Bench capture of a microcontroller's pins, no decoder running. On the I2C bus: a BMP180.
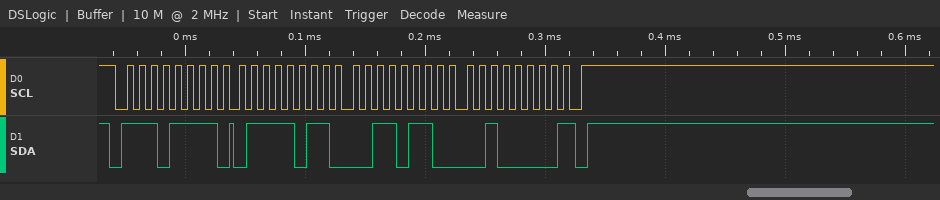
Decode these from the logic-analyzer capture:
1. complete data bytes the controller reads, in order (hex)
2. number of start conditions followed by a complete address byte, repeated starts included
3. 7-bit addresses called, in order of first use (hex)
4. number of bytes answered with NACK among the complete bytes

7B 36 20
1
0x77
1
